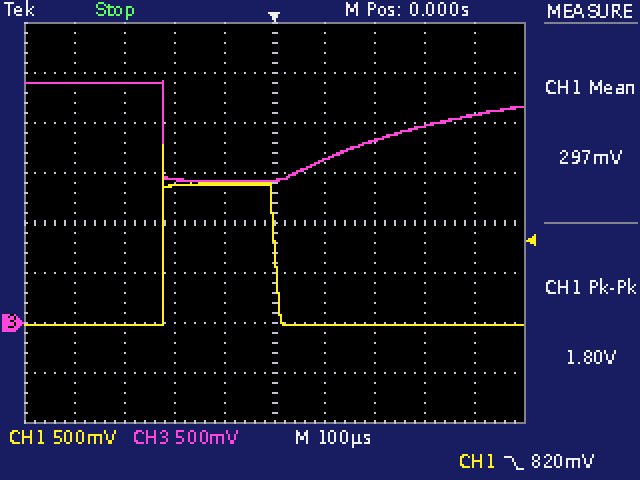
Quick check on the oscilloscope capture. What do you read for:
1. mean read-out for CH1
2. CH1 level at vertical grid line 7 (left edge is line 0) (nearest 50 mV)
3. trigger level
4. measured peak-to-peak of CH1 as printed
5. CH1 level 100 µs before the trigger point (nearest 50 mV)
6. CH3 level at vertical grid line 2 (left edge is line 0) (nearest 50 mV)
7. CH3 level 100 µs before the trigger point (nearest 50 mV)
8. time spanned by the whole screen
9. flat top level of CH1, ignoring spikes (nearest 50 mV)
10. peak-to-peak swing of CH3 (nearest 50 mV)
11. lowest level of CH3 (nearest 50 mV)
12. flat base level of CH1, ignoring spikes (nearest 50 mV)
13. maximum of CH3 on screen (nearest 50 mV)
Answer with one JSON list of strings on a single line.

["297 mV", "0 mV", "820 mV", "1.80 V", "1.40 V", "2.40 V", "1.40 V", "1 ms", "1.40 V", "1.00 V", "1.40 V", "0 mV", "2.40 V"]
